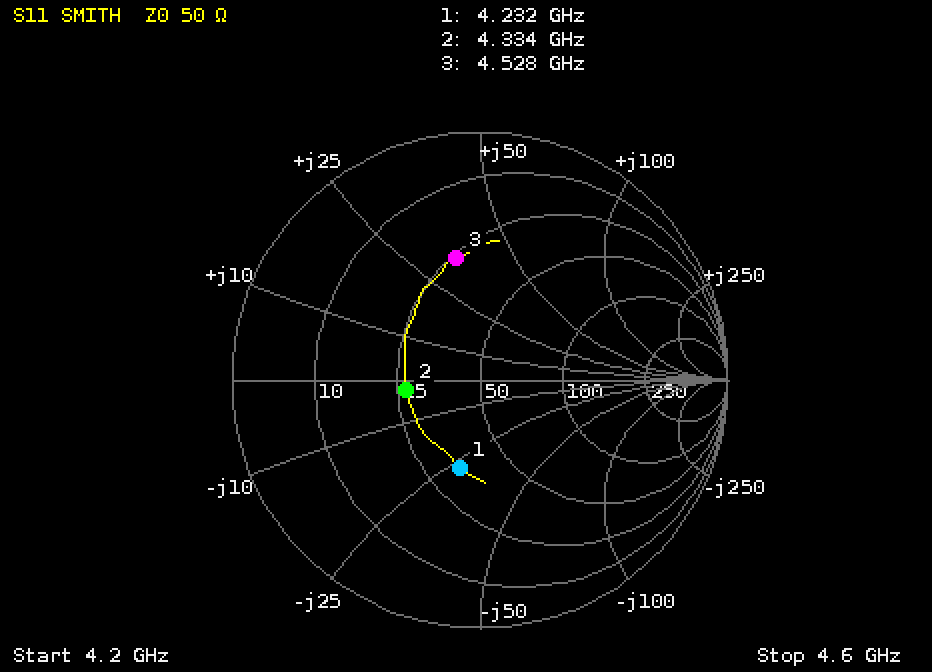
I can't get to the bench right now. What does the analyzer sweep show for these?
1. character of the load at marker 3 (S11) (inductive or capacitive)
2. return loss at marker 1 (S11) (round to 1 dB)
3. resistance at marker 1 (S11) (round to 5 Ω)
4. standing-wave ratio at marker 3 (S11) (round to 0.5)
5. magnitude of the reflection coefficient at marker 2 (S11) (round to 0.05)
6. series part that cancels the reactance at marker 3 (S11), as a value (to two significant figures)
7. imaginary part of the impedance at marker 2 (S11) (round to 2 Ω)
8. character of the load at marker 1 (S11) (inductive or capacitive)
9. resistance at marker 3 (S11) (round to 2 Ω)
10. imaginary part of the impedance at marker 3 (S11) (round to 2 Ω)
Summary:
inductive
9 dB
35 Ω
3.0
0.30
1.0 pF
-2 Ω
capacitive
26 Ω
+34 Ω
